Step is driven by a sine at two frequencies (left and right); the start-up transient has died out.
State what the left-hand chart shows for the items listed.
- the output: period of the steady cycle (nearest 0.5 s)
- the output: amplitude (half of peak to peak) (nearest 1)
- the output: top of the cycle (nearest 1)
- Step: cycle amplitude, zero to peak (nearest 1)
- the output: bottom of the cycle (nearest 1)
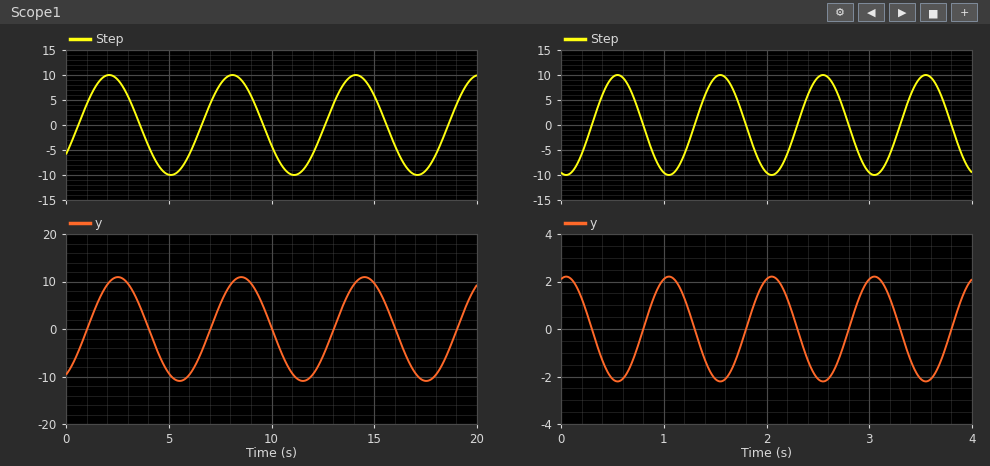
6.0 s
11
11
10
-11
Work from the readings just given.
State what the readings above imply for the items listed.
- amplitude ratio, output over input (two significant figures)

1.1
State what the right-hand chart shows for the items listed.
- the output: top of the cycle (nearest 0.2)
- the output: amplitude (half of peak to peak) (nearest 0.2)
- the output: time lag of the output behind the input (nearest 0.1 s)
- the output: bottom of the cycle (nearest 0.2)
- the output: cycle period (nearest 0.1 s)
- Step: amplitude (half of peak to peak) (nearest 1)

2.2
2.2
0.5 s
-2.2
1.0 s
10
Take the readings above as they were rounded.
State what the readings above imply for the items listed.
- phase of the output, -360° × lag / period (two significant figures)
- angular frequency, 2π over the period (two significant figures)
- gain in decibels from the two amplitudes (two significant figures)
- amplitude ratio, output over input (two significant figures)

-180°
6.3 rad/s
-13 dB
0.22
